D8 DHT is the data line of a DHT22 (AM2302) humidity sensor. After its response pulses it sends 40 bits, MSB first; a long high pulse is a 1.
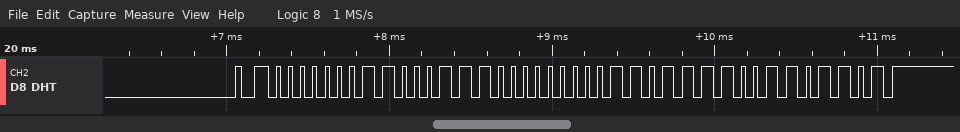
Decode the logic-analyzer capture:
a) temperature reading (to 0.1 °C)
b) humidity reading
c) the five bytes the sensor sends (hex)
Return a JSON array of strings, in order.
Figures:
["22.2 °C", "39.8 %", "01 8E 00 DE 6D"]
